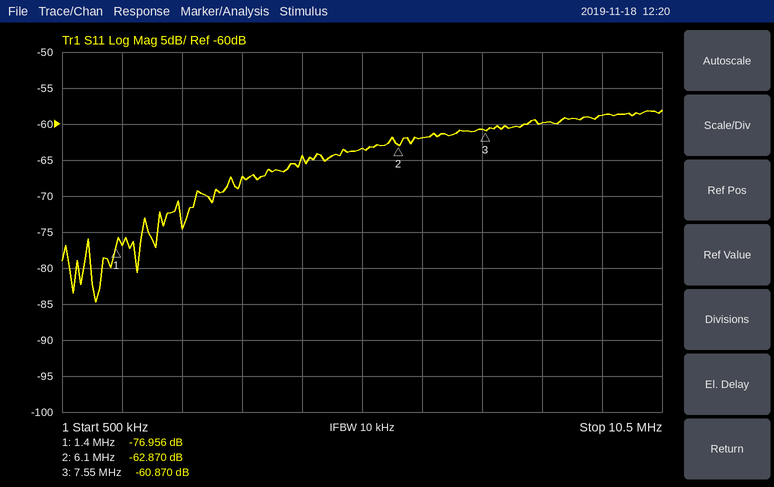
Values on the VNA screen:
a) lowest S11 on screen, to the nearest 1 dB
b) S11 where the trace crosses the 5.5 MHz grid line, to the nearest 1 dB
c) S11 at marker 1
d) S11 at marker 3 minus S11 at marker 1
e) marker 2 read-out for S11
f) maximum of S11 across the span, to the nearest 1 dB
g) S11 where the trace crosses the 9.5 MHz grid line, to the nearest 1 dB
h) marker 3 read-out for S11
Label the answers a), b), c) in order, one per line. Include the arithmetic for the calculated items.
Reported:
a) -85 dB
b) -63 dB
c) -76.956 dB
d) -60.87 − (-76.956) = 16.086 dB
e) -62.870 dB
f) -58 dB
g) -59 dB
h) -60.870 dB
